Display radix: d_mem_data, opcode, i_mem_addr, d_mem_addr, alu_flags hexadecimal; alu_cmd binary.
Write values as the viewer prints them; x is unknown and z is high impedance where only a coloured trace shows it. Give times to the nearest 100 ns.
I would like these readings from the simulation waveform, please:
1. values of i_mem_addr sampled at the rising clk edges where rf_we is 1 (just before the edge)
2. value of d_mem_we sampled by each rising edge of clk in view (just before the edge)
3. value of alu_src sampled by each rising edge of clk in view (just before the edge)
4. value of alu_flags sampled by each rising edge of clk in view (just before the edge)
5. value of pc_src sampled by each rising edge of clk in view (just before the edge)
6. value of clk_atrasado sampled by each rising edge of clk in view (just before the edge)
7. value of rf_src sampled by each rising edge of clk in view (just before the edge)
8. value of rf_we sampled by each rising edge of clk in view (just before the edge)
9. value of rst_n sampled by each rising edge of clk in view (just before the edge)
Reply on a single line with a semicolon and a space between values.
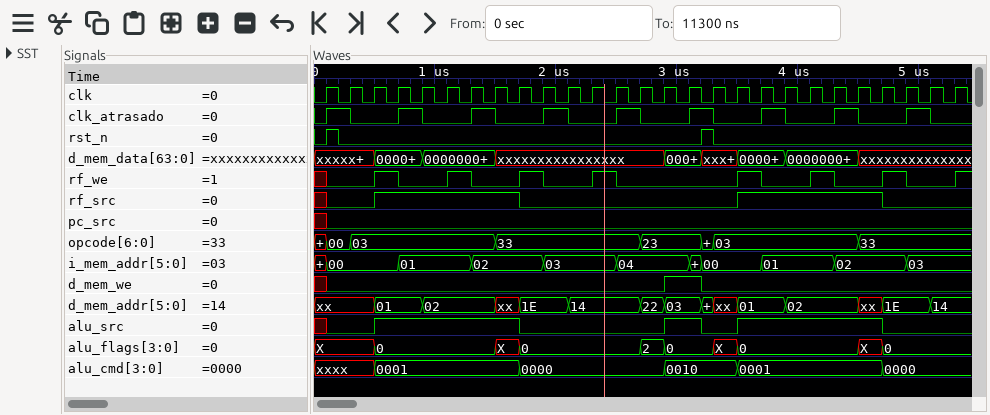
00, 01, 02, 03, 00, 01, 02; x 0 0 0 0 0 0 0 0 0 0 0 0 0 0 1 0 0 0 0 0 0 0 0 0 0 0; x 0 0 1 1 1 1 1 1 0 0 0 0 0 0 1 0 0 1 1 1 1 1 1 0 0 0; X, X, X, 0, 0, 0, 0, 0, X, 0, 0, 0, 0, 0, 2, 0, 0, X, 0, 0, 0, 0, 0, X, 0, 0, 0; x 0 0 0 0 0 0 0 0 0 0 0 0 0 0 0 0 0 0 0 0 0 0 0 0 0 0; 0 1 0 0 1 0 0 1 0 0 1 0 0 1 0 0 1 0 0 1 0 0 1 0 0 1 0; x 0 0 1 1 1 1 1 1 0 0 0 0 0 0 0 0 0 1 1 1 1 1 1 0 0 0; x 0 0 1 0 0 1 0 0 1 0 0 1 0 0 0 0 0 1 0 0 1 0 0 1 0 0; 0 0 0 0 0 0 0 0 0 0 0 0 0 0 0 0 1 0 0 0 0 0 0 0 0 0 0
